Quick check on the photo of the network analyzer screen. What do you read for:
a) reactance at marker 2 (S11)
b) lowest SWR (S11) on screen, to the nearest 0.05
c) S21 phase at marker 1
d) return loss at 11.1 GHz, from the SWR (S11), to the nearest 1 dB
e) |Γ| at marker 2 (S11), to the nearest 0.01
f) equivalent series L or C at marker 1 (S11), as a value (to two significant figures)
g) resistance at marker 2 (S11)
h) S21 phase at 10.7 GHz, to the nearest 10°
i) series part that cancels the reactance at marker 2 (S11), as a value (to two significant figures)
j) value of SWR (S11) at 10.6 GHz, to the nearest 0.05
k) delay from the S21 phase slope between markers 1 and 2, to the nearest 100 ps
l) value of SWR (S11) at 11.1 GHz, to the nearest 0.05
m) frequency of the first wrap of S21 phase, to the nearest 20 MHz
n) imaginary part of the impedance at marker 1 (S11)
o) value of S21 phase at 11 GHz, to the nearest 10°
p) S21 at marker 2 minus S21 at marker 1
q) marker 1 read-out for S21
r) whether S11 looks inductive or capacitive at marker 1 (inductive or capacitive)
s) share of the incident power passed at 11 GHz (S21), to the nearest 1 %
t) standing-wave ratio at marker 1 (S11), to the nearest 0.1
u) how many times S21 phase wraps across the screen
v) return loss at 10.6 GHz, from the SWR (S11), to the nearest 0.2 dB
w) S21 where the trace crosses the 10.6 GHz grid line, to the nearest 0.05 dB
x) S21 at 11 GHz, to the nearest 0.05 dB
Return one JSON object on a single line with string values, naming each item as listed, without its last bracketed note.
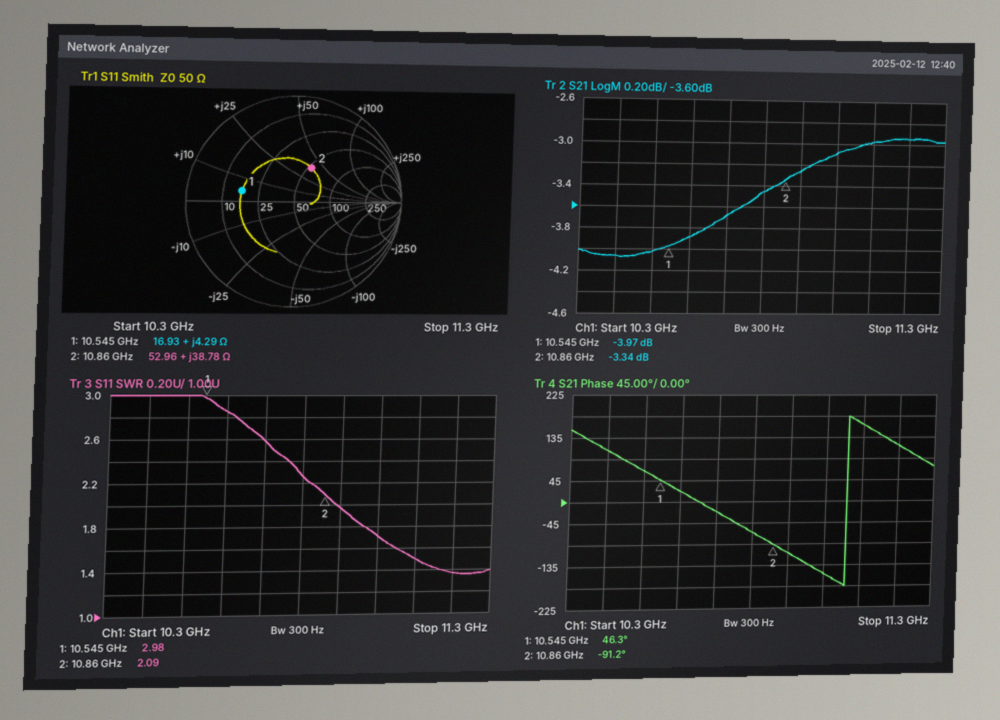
{"reactance at marker 2": "+38.78 Ω", "lowest SWR (S11) on screen, to the nearest 0.05": "1.35", "S21 phase at marker 1": "46.3°", "return loss at 11.1 GHz, from the SWR (S11), to the nearest 1 dB": "14 dB", "|Γ| at marker 2 (S11), to the nearest 0.01": "0.35", "equivalent series L or C at marker 1 (S11), as a value": "65 pH", "resistance at marker 2": "52.96 Ω", "S21 phase at 10.7 GHz, to the nearest 10°": "-20°", "series part that cancels the reactance at marker 2 (S11), as a value": "380 fF", "value of SWR (S11) at 10.6 GHz, to the nearest 0.05": "2.85", "delay from the S21 phase slope between markers 1 and 2, to the nearest 100 ps": "1.2 ns", "value of SWR (S11) at 11.1 GHz, to the nearest 0.05": "1.50", "frequency of the first wrap of S21 phase, to the nearest 20 MHz": "11.06 GHz", "imaginary part of the impedance at marker 1": "+4.29 Ω", "value of S21 phase at 11 GHz, to the nearest 10°": "-150°", "S21 at marker 2 minus S21 at marker 1": "0.63 dB", "marker 1 read-out for S21": "-3.97 dB", "whether S11 looks inductive or capacitive at marker 1": "inductive", "share of the incident power passed at 11 GHz (S21), to the nearest 1 %": "49 %", "standing-wave ratio at marker 1 (S11), to the nearest 0.1": "3.0", "how many times S21 phase wraps across the screen": "1", "return loss at 10.6 GHz, from the SWR (S11), to the nearest 0.2 dB": "6.4 dB", "S21 where the trace crosses the 10.6 GHz grid line, to the nearest 0.05 dB": "-3.90 dB", "S21 at 11 GHz, to the nearest 0.05 dB": "-3.10 dB"}
